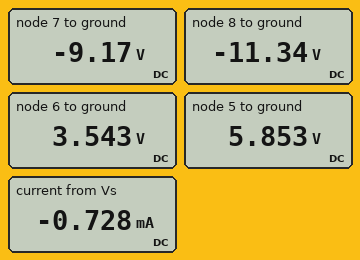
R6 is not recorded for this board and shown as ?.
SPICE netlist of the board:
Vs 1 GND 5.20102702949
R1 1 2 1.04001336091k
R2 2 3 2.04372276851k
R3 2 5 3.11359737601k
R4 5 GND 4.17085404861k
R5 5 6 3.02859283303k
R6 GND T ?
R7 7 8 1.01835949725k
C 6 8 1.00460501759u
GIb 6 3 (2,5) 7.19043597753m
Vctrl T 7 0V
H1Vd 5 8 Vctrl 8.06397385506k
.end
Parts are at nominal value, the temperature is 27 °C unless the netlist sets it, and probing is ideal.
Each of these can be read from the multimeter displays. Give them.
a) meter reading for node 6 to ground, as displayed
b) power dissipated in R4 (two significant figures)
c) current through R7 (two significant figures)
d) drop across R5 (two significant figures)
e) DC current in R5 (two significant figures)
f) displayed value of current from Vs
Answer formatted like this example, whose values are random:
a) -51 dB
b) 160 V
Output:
a) 3.543 V
b) 8.2 mW
c) 2.1 mA
d) 2.3 V
e) 760 µA
f) -0.728 mA
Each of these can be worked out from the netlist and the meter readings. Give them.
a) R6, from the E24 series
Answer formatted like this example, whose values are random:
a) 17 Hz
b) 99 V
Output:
a) 4.3 kΩ
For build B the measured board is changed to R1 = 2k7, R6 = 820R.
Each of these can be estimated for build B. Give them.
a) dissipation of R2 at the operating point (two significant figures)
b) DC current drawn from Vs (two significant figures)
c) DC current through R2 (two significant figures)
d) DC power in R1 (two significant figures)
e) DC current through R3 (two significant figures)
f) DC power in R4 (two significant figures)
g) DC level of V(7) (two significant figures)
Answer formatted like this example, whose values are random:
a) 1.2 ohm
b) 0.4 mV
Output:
a) 260 µW
b) 340 µA
c) 360 µA
d) 320 µW
e) 16 µA
f) 4.5 mW
g) -570 mV
